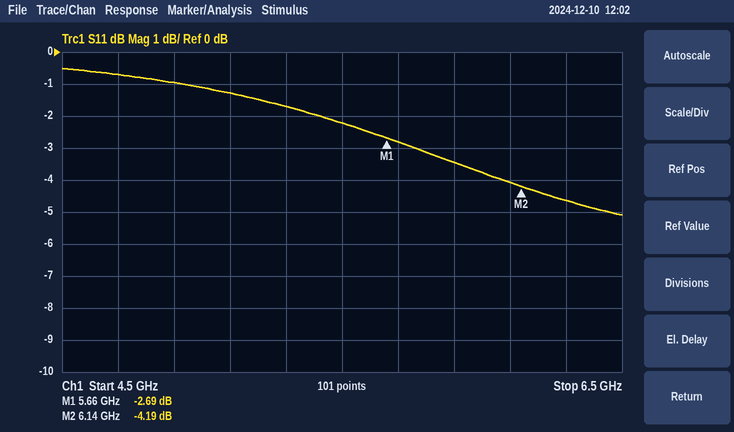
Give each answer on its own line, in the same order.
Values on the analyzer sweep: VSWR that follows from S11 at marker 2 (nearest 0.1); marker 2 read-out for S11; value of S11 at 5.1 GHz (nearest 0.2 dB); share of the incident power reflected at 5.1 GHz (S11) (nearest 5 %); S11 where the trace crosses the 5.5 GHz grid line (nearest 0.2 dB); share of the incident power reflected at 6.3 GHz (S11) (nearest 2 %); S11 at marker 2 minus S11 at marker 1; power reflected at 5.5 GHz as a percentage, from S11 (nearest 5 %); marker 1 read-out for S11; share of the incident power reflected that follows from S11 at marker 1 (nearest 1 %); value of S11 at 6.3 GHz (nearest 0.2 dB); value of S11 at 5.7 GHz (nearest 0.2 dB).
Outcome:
4.2
-4.19 dB
-1.2 dB
75 %
-2.2 dB
34 %
-1.50 dB
60 %
-2.69 dB
54 %
-4.6 dB
-2.8 dB
